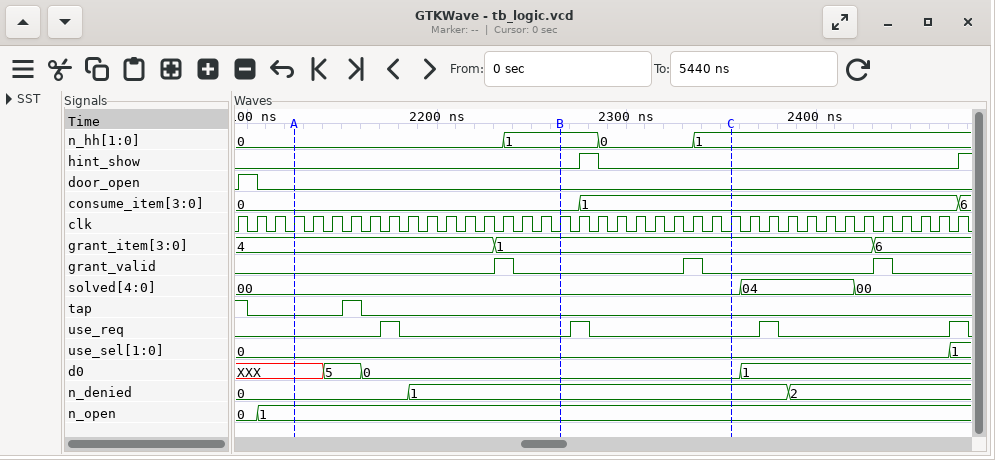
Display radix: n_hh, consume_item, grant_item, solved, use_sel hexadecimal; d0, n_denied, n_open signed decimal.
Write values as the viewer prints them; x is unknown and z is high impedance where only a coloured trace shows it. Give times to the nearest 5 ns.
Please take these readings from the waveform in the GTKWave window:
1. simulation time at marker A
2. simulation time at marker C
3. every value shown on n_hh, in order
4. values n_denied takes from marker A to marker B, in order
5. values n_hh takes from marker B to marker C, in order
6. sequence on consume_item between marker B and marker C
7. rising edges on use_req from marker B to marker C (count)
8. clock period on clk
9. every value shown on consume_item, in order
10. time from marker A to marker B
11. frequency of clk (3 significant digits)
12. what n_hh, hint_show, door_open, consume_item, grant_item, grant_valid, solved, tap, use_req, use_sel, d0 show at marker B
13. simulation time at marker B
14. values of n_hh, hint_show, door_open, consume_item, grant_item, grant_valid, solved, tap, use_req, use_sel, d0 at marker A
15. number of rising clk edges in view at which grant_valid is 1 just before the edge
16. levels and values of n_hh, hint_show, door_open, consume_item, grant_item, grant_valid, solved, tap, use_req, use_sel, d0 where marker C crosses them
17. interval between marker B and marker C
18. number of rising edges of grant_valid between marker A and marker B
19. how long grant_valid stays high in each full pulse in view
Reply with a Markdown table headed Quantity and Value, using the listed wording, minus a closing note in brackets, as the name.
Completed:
| Quantity | Value |
|---|---|
| simulation time at marker A | 2125 ns |
| simulation time at marker C | 2355 ns |
| every value shown on n_hh, in order | 0, 1, 0, 1 |
| values n_denied takes from marker A to marker B, in order | 0, 1 |
| values n_hh takes from marker B to marker C, in order | 1, 0, 1 |
| sequence on consume_item between marker B and marker C | 0, 1 |
| rising edges on use_req from marker B to marker C | 1 |
| clock period on clk | 10 ns |
| every value shown on consume_item, in order | 0, 1, 6 |
| time from marker A to marker B | 140 ns |
| frequency of clk | 100 MHz |
| what n_hh, hint_show, door_open, consume_item, grant_item, grant_valid, solved, tap, use_req, use_sel, d0 show at marker B | n_hh=1, hint_show=0, door_open=0, consume_item=0, grant_item=1, grant_valid=0, solved=00, tap=0, use_req=0, use_sel=0, d0=0 |
| simulation time at marker B | 2265 ns |
| values of n_hh, hint_show, door_open, consume_item, grant_item, grant_valid, solved, tap, use_req, use_sel, d0 at marker A | n_hh=0, hint_show=0, door_open=0, consume_item=0, grant_item=4, grant_valid=0, solved=00, tap=0, use_req=0, use_sel=0, d0=XXX |
| number of rising clk edges in view at which grant_valid is 1 just before the edge | 3 |
| levels and values of n_hh, hint_show, door_open, consume_item, grant_item, grant_valid, solved, tap, use_req, use_sel, d0 where marker C crosses them | n_hh=1, hint_show=0, door_open=0, consume_item=1, grant_item=1, grant_valid=0, solved=00, tap=0, use_req=0, use_sel=0, d0=0 |
| interval between marker B and marker C | 90 ns |
| number of rising edges of grant_valid between marker A and marker B | 1 |
| how long grant_valid stays high in each full pulse in view | 10 ns, 10 ns, 10 ns |
